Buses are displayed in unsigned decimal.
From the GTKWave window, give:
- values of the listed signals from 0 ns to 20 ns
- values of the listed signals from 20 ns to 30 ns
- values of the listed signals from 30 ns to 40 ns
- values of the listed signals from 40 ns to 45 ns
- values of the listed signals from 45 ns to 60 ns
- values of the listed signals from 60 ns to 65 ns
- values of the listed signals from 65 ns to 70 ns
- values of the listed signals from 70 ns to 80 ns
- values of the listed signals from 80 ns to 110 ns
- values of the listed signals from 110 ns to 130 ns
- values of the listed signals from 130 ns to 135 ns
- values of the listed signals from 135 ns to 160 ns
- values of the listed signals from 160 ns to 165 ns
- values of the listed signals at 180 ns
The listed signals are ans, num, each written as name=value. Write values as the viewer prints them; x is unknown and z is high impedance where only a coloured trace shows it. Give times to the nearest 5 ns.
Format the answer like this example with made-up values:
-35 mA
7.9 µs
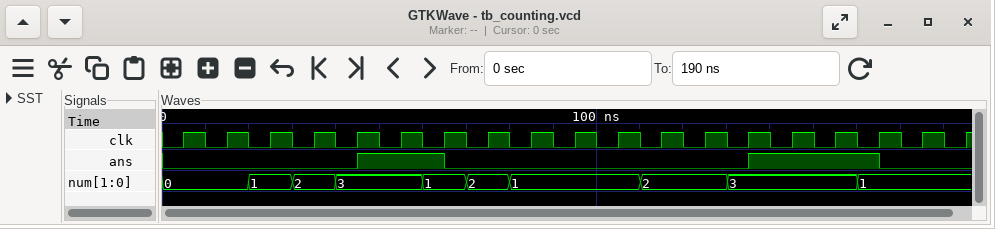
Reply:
ans=0, num=0
ans=0, num=1
ans=0, num=2
ans=0, num=3
ans=1, num=3
ans=1, num=1
ans=0, num=1
ans=0, num=2
ans=0, num=1
ans=0, num=2
ans=0, num=3
ans=1, num=3
ans=1, num=1
ans=0, num=1
